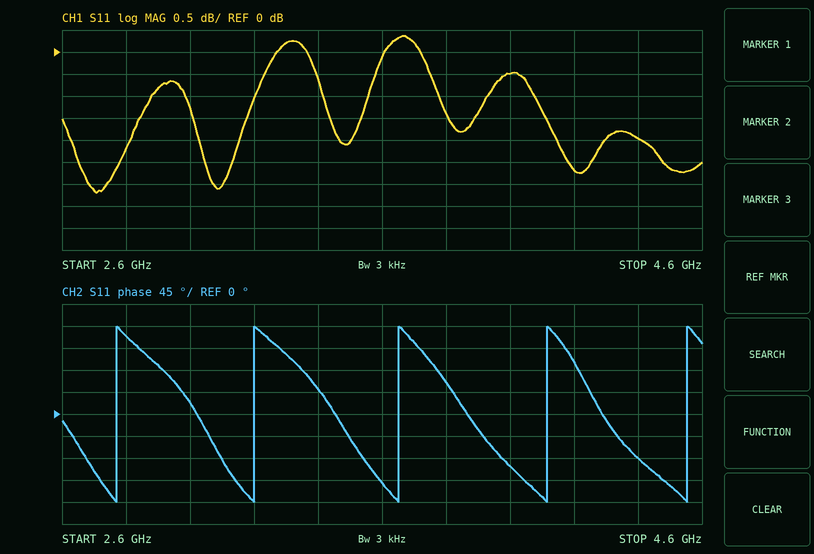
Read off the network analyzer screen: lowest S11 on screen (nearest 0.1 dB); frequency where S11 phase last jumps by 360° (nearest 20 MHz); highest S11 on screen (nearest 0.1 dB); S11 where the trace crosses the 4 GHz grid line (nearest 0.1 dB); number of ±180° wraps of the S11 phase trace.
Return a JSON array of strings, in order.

["-3.2 dB", "4.56 GHz", "0.4 dB", "-0.5 dB", "5"]
